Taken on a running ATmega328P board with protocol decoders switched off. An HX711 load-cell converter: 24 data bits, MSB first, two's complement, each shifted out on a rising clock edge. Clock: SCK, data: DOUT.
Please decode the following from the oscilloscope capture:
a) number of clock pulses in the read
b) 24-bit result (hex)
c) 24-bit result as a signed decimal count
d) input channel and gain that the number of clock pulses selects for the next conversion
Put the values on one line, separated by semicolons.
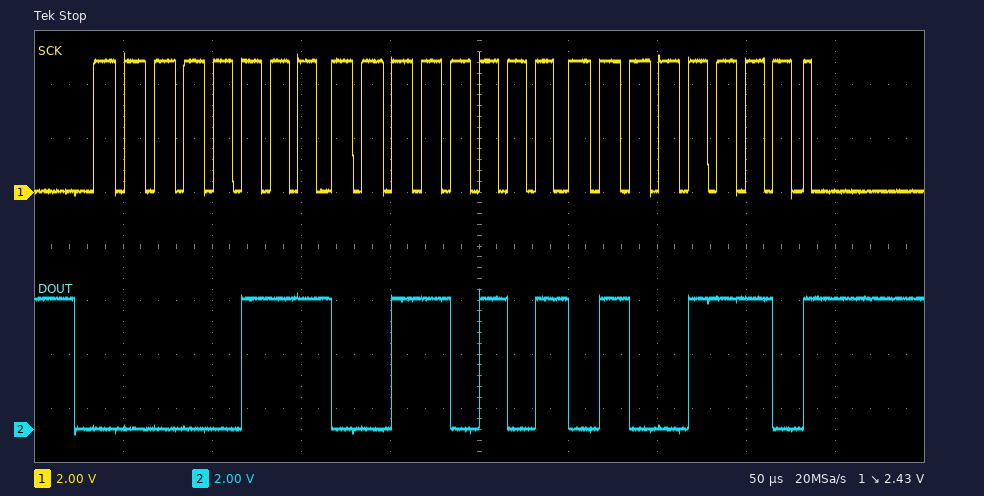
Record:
25; 0x07354E; 472398; channel A, gain 128
